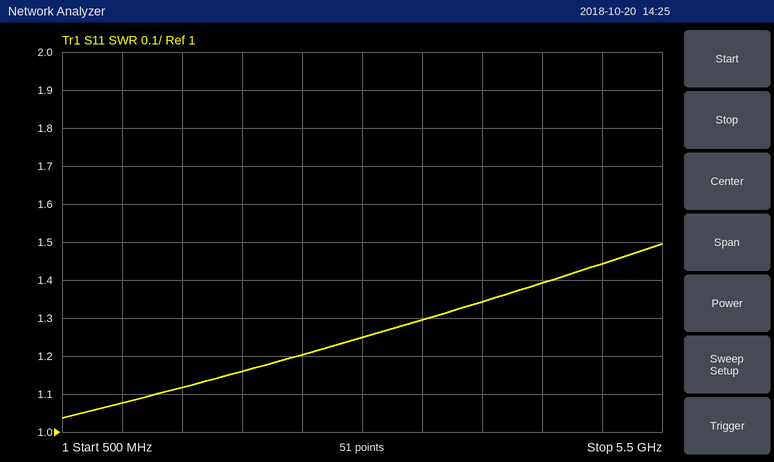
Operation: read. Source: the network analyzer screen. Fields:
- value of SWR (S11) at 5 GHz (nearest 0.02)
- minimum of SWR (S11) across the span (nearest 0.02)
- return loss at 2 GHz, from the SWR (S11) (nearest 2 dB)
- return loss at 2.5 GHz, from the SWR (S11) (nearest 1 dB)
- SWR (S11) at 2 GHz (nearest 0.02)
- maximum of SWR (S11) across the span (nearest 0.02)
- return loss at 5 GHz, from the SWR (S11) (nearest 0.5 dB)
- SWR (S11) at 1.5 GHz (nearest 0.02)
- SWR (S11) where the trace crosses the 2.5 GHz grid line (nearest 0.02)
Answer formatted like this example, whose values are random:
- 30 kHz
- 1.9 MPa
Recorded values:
- 1.44
- 1.04
- 22 dB
- 21 dB
- 1.16
- 1.50
- 15.0 dB
- 1.12
- 1.20
